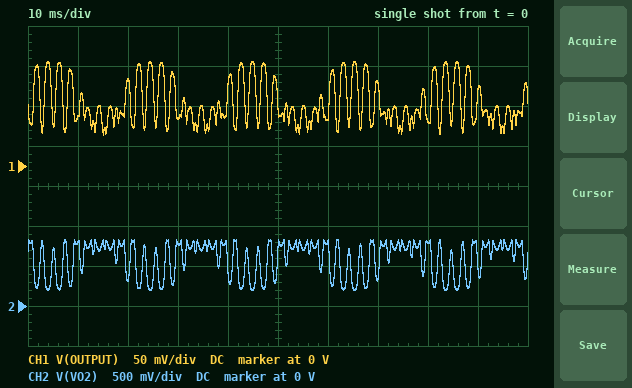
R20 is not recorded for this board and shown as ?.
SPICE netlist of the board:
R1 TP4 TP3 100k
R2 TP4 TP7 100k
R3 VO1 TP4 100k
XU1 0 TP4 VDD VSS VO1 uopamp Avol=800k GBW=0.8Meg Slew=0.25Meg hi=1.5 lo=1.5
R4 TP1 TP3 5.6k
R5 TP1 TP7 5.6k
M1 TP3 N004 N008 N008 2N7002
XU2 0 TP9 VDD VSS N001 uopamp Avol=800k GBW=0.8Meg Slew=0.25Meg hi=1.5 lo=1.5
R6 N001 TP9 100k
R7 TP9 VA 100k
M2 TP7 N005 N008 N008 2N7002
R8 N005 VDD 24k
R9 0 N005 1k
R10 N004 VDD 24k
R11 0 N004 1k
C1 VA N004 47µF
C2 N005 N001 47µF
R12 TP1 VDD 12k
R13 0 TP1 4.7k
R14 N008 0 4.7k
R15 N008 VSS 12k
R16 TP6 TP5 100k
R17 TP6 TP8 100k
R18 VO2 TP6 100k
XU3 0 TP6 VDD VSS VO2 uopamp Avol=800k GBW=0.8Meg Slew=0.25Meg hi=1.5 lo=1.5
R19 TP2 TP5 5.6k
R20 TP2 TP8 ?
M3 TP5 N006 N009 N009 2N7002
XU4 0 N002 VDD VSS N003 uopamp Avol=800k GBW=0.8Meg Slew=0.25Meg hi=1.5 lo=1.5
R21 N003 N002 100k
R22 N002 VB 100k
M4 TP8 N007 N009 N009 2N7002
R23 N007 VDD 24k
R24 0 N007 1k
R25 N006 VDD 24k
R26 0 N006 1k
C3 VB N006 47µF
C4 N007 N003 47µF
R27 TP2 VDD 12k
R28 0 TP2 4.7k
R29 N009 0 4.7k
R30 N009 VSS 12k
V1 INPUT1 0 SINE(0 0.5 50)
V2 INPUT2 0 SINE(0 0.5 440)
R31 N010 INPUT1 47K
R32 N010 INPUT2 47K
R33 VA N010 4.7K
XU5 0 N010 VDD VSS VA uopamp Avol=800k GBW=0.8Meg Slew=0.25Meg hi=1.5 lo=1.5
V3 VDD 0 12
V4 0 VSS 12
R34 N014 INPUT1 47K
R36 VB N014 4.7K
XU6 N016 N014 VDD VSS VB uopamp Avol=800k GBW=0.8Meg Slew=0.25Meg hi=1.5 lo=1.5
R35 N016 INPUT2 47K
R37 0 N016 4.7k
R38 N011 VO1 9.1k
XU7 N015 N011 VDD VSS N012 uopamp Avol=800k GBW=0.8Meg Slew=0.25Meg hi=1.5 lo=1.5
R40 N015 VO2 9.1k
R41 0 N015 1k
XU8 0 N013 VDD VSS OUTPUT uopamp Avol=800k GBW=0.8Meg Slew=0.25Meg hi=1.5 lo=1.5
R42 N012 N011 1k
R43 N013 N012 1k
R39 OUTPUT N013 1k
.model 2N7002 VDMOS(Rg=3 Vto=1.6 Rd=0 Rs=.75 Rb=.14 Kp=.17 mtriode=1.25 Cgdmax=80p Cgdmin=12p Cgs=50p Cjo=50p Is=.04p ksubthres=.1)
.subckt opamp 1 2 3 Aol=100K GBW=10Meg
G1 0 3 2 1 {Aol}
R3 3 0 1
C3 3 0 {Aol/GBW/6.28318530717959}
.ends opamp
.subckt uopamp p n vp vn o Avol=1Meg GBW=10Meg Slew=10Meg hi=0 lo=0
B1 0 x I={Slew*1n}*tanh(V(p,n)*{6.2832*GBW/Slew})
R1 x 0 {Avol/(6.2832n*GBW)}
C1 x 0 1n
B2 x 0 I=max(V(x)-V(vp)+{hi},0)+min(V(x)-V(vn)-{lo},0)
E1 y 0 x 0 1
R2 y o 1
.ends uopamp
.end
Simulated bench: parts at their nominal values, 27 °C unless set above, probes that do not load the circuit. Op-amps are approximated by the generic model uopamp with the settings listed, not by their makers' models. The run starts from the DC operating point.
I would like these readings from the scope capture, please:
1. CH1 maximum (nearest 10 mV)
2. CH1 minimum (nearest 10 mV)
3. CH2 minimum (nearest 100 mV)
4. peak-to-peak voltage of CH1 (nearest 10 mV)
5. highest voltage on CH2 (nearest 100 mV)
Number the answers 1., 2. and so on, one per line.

1. 130 mV
2. 40 mV
3. 200 mV
4. 90 mV
5. 800 mV
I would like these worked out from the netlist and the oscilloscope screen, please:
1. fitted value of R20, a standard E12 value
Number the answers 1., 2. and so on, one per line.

1. 3.3 kΩ
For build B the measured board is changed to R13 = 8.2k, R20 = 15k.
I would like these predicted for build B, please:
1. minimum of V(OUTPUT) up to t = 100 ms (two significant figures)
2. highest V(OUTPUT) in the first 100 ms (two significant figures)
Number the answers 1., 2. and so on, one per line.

1. -230 mV
2. -210 mV
